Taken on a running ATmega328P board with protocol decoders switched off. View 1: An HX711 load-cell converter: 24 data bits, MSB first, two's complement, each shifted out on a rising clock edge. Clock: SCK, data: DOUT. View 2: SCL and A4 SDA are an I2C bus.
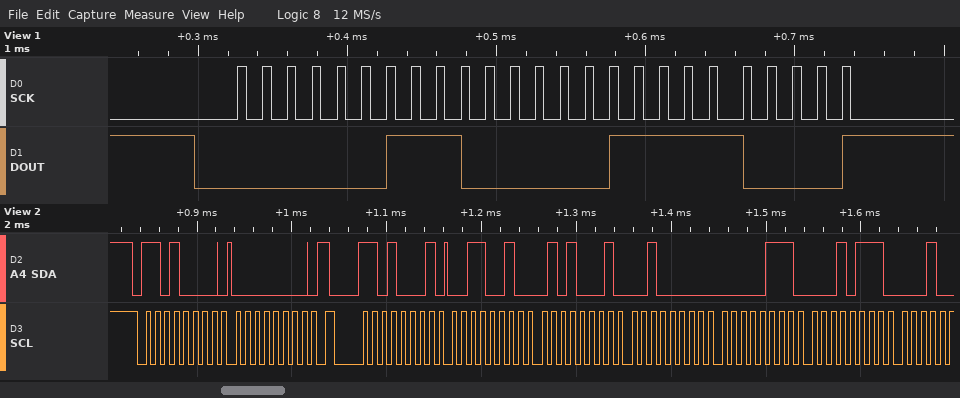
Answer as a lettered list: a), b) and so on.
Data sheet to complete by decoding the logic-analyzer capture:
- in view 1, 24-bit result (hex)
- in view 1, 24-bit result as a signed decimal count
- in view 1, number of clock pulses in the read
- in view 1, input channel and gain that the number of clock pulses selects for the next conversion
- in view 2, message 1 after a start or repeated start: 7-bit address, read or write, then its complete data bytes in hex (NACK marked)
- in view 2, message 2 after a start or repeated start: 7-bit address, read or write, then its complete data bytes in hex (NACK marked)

a) 0x0381F0
b) 229872
c) 25
d) channel A, gain 128
e) 0x68 write: 00
f) 0x68 read: 32 51 20 07 17
